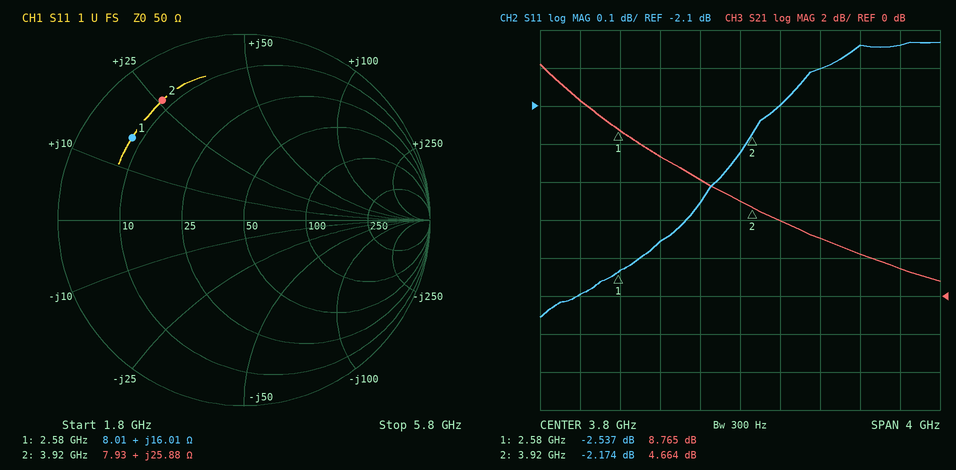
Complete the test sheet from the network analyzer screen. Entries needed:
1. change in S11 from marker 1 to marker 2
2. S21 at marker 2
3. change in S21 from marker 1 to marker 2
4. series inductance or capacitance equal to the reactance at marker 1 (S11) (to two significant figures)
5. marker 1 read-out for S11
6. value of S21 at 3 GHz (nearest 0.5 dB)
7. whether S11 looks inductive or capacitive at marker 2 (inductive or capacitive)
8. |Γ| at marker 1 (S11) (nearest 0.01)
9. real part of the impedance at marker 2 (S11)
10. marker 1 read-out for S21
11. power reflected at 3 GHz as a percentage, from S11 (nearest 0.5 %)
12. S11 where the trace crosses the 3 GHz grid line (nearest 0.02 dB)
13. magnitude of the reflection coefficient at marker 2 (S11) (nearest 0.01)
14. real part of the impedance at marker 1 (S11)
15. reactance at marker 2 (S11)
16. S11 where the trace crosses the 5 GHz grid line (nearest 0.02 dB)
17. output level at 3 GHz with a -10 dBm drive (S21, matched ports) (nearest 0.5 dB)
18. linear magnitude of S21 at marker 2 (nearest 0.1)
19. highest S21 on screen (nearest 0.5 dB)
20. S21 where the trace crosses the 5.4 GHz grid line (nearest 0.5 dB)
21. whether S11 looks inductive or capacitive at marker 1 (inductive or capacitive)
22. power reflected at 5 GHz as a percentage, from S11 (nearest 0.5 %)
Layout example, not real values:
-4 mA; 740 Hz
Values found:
0.363 dB; 4.664 dB; -4.101 dB; 990 pH; -2.537 dB; 7.5 dB; inductive; 0.75; 7.93 Ω; 8.765 dB; 57.0 %; -2.46 dB; 0.78; 8.01 Ω; +25.88 Ω; -1.94 dB; -2.5 dBm; 1.7; 12.0 dB; 1.5 dB; inductive; 64.0 %
